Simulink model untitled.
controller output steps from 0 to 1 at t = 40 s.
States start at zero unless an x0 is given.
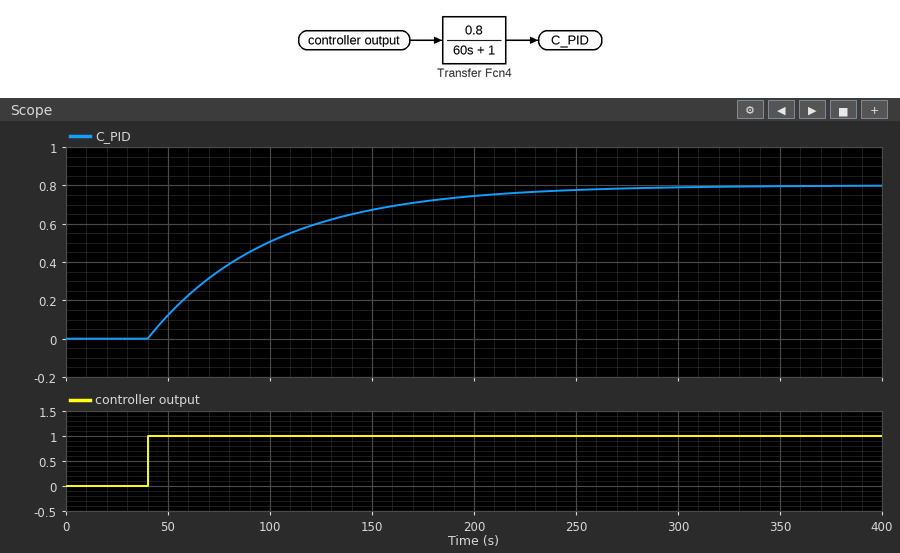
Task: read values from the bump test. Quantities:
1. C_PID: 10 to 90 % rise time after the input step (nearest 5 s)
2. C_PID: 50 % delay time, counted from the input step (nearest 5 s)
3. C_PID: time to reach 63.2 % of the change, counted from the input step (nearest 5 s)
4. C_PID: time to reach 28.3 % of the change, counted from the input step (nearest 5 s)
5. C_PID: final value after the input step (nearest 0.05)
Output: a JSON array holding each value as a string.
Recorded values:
["130 s", "40 s", "60 s", "20 s", "0.80"]
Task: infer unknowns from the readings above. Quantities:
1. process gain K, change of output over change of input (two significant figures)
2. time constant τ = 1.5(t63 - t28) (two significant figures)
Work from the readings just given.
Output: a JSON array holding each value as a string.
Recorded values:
["0.80", "60 s"]
